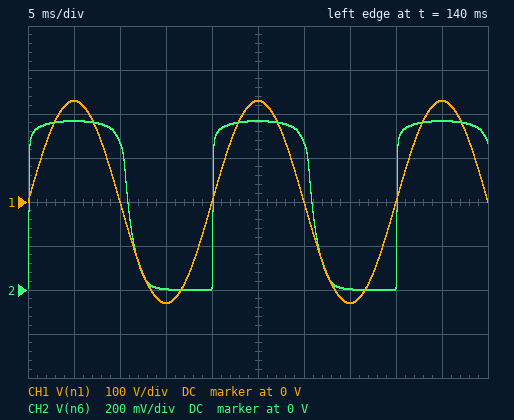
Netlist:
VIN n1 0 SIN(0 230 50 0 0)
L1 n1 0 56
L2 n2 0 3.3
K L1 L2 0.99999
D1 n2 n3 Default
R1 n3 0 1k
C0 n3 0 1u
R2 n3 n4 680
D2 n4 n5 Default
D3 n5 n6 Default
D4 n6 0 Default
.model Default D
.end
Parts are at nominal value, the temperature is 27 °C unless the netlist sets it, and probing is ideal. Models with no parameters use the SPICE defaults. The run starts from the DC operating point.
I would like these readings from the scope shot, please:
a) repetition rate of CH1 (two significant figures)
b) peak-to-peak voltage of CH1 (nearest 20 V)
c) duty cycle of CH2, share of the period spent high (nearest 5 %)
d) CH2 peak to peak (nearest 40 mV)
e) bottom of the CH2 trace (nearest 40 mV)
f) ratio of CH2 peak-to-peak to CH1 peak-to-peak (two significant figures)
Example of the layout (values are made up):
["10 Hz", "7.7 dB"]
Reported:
["50 Hz", "460 V", "55 %", "760 mV", "0 V", "0.0017"]
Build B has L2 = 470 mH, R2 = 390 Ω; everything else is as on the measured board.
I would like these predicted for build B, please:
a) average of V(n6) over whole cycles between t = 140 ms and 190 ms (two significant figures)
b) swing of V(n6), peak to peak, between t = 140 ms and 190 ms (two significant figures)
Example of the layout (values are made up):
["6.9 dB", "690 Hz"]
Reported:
["380 mV", "750 mV"]
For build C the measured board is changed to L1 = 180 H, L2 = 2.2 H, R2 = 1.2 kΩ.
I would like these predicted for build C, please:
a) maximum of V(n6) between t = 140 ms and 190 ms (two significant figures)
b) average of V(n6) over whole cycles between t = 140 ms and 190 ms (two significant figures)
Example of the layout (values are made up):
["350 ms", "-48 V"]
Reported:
["730 mV", "380 mV"]
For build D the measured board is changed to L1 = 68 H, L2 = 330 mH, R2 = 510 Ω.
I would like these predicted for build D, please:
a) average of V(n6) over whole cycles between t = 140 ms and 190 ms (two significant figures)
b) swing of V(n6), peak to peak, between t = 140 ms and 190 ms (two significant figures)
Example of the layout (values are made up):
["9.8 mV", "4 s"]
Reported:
["360 mV", "740 mV"]
